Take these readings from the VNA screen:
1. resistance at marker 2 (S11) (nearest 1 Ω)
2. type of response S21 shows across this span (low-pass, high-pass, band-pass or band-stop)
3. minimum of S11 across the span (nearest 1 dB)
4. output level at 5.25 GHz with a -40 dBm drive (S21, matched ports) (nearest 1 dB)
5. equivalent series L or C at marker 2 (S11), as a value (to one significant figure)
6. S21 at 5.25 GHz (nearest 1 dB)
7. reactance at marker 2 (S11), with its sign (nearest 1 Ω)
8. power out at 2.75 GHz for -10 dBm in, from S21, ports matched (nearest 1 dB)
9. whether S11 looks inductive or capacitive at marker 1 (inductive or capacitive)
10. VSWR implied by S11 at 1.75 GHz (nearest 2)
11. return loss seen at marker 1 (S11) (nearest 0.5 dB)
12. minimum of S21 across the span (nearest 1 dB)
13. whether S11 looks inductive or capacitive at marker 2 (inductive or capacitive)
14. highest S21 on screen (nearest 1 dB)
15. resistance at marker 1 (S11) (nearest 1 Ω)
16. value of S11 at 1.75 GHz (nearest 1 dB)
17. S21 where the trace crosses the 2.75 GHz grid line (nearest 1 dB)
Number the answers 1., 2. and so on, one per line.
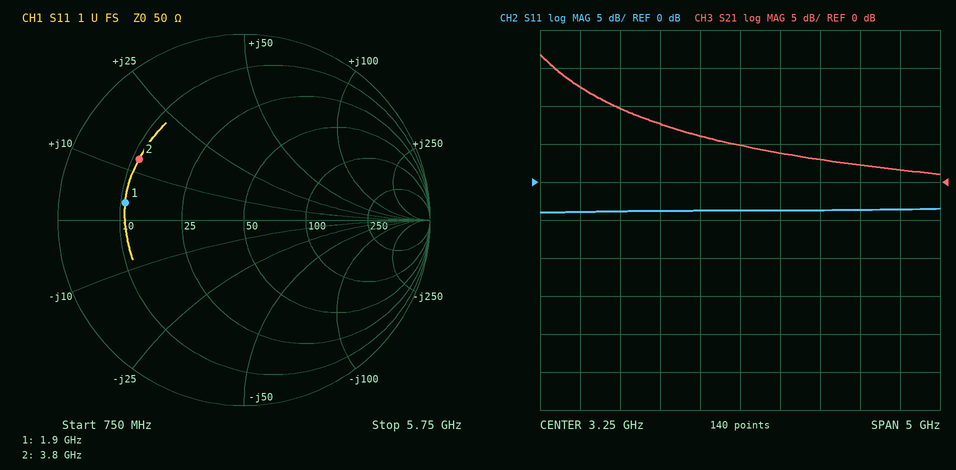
1. 11 Ω
2. low-pass
3. -4 dB
4. -38 dBm
5. 500 pH
6. 2 dB
7. +13 Ω
8. -4 dBm
9. inductive
10. 4
11. 4.0 dB
12. 1 dB
13. inductive
14. 17 dB
15. 11 Ω
16. -4 dB
17. 6 dB
